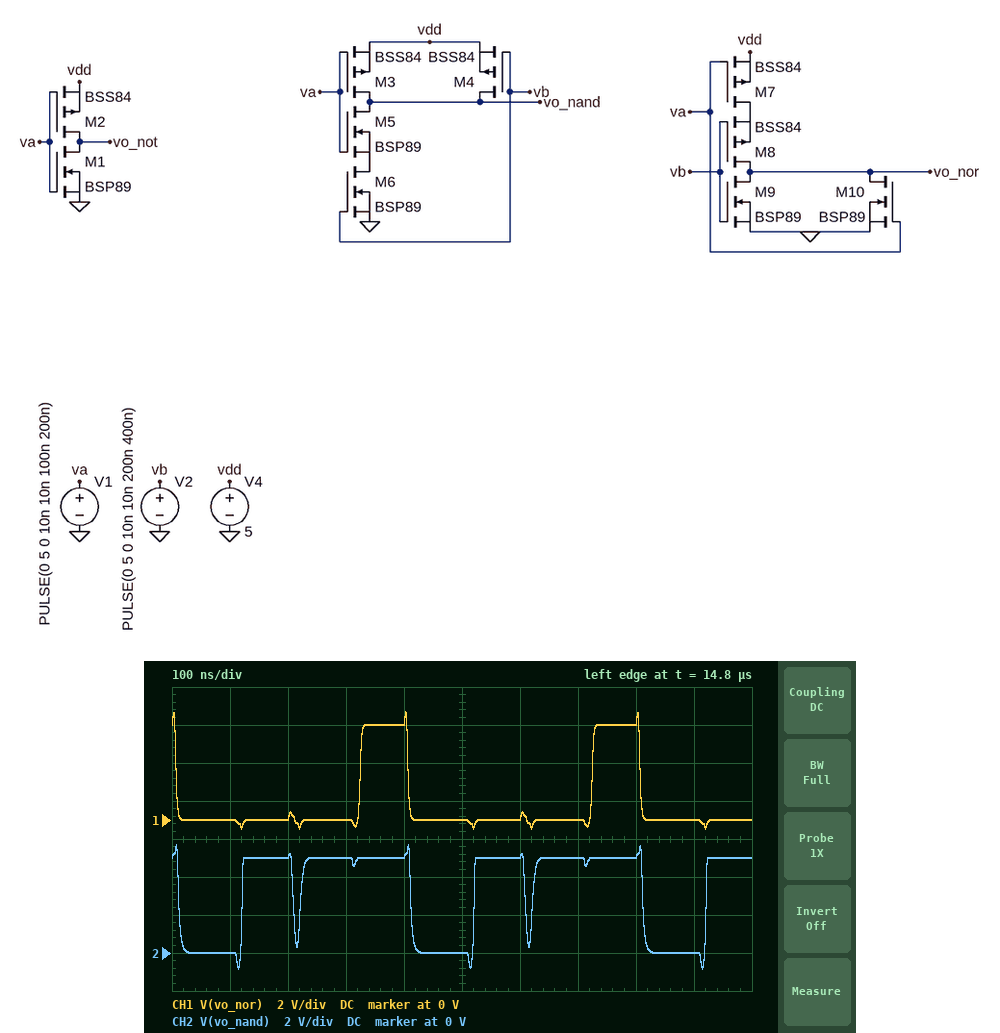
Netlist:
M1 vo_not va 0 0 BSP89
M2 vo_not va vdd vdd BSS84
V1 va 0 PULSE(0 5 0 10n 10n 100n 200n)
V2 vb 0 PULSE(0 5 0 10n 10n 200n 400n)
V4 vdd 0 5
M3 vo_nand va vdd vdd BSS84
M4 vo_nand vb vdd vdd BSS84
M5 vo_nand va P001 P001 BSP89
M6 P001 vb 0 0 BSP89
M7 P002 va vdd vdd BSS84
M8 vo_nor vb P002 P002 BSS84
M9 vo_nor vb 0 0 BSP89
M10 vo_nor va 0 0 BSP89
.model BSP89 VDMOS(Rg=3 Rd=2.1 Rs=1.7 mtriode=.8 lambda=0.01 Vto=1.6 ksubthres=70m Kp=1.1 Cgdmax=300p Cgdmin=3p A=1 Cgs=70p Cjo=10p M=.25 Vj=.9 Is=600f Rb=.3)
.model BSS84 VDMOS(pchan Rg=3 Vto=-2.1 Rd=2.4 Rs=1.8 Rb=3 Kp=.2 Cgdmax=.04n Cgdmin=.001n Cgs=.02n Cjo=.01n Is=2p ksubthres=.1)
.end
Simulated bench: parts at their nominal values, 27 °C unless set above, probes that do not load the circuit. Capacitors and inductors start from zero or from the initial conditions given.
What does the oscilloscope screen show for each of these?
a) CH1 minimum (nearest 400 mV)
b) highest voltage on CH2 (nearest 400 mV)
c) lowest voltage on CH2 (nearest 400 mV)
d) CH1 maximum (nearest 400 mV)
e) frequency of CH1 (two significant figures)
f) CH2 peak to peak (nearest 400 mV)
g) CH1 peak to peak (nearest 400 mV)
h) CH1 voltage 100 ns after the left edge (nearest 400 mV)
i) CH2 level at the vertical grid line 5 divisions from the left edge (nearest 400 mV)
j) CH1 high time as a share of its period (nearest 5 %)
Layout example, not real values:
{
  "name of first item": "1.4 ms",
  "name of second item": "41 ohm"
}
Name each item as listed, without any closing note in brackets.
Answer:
{
  "CH1 minimum": "-400 mV",
  "highest voltage on CH2": "5.6 V",
  "lowest voltage on CH2": "-800 mV",
  "CH1 maximum": "5.6 V",
  "frequency of CH1": "2.5 MHz",
  "CH2 peak to peak": "6.4 V",
  "CH1 peak to peak": "6.0 V",
  "CH1 voltage 100 ns after the left edge": "0 V",
  "CH2 level at the vertical grid line 5 divisions from the left edge": "0 V",
  "CH1 high time as a share of its period": "20 %"
}
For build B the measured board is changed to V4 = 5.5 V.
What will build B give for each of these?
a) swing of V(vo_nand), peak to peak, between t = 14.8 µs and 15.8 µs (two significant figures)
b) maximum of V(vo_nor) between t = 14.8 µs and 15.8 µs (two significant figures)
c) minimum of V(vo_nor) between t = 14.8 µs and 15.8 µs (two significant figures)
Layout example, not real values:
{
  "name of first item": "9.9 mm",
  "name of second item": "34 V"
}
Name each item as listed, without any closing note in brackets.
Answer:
{
  "swing of V(vo_nand), peak to peak, between t = 14.8 µs and 15.8 µs": "6.8 V",
  "maximum of V(vo_nor) between t = 14.8 µs and 15.8 µs": "6.1 V",
  "minimum of V(vo_nor) between t = 14.8 µs and 15.8 µs": "-460 mV"
}
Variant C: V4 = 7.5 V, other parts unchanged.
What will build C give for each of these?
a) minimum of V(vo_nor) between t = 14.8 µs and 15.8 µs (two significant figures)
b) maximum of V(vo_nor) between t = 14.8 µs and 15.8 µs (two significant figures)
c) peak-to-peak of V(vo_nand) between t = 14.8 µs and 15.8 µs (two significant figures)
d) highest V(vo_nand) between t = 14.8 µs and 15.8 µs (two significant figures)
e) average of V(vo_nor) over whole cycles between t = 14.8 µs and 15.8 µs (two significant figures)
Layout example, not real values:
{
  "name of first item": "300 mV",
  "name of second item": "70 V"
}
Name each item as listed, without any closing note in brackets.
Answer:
{
  "minimum of V(vo_nor) between t = 14.8 µs and 15.8 µs": "-430 mV",
  "maximum of V(vo_nor) between t = 14.8 µs and 15.8 µs": "8.0 V",
  "peak-to-peak of V(vo_nand) between t = 14.8 µs and 15.8 µs": "7.5 V",
  "highest V(vo_nand) between t = 14.8 µs and 15.8 µs": "7.6 V",
  "average of V(vo_nor) over whole cycles between t = 14.8 µs and 15.8 µs": "1.7 V"
}
